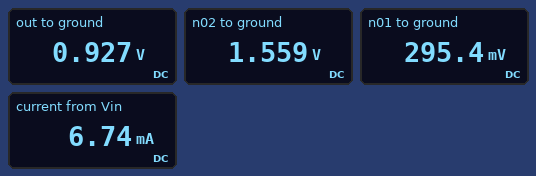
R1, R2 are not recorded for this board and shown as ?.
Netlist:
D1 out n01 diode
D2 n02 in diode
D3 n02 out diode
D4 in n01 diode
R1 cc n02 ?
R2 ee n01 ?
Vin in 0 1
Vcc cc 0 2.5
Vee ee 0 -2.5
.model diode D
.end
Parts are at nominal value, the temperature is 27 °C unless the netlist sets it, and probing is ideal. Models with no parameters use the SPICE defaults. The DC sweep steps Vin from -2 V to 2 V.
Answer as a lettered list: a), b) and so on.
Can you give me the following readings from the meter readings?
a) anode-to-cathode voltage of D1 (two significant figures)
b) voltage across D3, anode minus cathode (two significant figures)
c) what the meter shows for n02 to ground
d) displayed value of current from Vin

a) 630 mV
b) 630 mV
c) 1.559 V
d) 6.74 mA
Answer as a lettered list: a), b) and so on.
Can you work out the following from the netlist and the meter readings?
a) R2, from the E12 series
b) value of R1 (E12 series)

a) 390 Ω
b) 2.2 kΩ
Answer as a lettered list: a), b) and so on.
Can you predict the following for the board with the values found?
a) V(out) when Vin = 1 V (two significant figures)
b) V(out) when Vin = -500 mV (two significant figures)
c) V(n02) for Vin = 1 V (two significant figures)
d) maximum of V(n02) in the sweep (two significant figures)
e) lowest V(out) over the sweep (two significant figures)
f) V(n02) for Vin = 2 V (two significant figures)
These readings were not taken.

a) 930 mV
b) -530 mV
c) 1.6 V
d) 2.4 V
e) -1.9 V
f) 2.4 V
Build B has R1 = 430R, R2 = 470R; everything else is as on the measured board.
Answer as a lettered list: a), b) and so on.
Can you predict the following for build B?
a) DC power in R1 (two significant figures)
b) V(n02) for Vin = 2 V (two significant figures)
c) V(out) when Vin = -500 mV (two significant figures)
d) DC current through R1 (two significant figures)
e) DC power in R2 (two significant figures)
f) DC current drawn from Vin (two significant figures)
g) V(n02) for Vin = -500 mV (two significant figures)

a) 1.7 mW
b) 2.5 V
c) -480 mV
d) 2.0 mA
e) 17 mW
f) 4.0 mA
g) 190 mV
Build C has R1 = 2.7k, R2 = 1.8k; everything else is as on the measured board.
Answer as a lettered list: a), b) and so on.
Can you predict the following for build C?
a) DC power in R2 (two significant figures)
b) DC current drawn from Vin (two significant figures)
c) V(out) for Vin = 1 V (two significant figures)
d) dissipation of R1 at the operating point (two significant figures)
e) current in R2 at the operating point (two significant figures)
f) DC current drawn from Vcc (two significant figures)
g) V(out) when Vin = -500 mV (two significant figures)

a) 4.5 mW
b) 1.2 mA
c) 960 mV
d) 310 µW
e) 1.6 mA
f) 340 µA
g) -500 mV
